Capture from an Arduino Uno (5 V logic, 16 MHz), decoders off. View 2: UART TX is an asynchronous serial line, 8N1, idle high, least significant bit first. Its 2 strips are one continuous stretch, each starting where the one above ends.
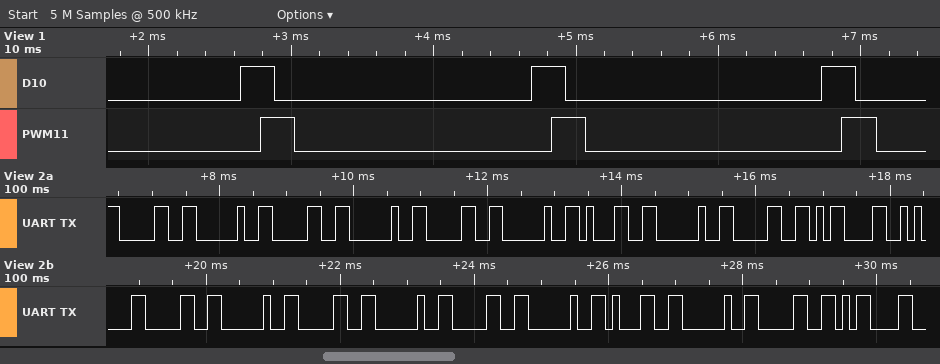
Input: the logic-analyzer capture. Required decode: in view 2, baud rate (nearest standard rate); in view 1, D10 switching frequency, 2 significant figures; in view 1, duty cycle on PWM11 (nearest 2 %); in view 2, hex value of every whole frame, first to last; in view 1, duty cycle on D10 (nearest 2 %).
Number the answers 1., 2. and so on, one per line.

1. 9600 baud
2. 490 Hz
3. 12 %
4. 30 20 30 20 30 20 31 20 30 0D 0A 30 20 30 20 30 20 31 20 30 0D
5. 12 %
